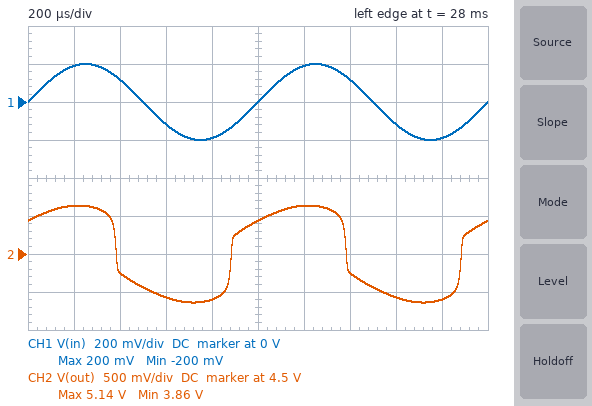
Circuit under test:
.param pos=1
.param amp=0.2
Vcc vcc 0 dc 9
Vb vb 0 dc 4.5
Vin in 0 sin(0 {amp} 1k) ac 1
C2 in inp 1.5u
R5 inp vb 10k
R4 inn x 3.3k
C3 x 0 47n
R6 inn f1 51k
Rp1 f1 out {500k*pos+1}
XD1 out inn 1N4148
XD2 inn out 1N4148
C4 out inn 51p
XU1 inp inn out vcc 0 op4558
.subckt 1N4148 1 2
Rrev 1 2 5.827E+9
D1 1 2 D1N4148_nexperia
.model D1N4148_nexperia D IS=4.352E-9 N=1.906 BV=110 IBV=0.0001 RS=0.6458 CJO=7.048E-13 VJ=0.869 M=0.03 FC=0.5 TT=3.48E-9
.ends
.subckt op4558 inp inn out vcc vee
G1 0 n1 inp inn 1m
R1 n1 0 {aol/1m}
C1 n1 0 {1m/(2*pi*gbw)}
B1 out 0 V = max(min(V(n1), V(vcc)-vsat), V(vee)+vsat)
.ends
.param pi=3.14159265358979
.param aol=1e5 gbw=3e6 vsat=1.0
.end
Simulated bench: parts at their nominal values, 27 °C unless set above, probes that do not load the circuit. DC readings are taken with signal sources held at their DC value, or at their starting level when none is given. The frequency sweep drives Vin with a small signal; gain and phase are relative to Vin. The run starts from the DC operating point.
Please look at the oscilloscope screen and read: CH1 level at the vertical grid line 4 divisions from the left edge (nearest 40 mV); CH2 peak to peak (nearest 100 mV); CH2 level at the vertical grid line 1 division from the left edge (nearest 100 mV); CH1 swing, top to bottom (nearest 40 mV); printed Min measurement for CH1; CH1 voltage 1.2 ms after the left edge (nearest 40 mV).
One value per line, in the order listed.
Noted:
-200 mV
1.3 V
5.1 V
400 mV
-200 mV
200 mV
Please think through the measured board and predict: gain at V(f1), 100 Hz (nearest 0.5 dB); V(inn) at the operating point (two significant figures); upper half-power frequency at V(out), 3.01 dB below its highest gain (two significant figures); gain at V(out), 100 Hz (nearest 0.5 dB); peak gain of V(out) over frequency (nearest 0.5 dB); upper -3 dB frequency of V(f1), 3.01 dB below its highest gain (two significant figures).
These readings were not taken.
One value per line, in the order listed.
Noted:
5.0 dB
4.5 V
6.2 kHz
23.5 dB
42.5 dB
6.2 kHz
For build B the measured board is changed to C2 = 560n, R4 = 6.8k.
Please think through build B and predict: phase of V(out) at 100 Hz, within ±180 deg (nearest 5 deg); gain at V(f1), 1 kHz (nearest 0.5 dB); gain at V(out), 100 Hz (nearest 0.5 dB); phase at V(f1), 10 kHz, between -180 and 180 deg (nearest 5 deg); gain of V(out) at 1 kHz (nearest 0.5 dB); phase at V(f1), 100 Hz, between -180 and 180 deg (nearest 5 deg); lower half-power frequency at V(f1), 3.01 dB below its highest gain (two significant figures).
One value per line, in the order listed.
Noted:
90 deg
17.0 dB
23.0 dB
-50 deg
36.5 dB
60 deg
420 Hz
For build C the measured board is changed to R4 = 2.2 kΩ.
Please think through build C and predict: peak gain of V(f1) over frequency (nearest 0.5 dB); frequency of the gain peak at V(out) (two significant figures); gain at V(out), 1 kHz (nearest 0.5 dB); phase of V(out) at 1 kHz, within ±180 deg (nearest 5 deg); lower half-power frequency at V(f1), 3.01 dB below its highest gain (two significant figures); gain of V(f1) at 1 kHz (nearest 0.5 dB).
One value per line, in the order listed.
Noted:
25.0 dB
2.5 kHz
42.0 dB
45 deg
1.0 kHz
22.0 dB
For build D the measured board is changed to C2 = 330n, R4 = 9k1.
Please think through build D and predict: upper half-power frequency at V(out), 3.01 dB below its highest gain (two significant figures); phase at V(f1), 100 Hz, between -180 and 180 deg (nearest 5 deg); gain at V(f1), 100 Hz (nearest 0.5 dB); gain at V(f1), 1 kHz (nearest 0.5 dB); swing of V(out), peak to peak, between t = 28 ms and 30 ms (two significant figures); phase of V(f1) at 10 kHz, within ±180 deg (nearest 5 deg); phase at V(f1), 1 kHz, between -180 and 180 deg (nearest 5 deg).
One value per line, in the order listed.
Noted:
6.1 kHz
70 deg
4.5 dB
15.0 dB
1.2 V
-45 deg
10 deg
